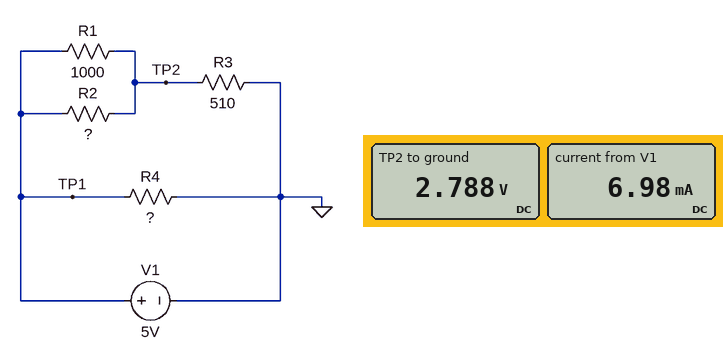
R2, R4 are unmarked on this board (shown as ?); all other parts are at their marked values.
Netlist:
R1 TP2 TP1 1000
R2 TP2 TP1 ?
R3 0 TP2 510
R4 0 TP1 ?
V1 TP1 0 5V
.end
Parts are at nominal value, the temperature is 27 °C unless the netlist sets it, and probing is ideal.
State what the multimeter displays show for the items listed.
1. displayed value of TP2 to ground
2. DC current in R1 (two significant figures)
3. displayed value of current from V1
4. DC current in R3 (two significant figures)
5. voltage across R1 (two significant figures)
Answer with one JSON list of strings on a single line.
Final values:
["2.788 V", "2.2 mA", "6.98 mA", "5.5 mA", "2.2 V"]
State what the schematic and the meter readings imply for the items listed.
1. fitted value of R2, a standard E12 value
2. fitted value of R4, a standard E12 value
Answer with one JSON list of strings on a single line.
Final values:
["680 Ω", "3.3 kΩ"]
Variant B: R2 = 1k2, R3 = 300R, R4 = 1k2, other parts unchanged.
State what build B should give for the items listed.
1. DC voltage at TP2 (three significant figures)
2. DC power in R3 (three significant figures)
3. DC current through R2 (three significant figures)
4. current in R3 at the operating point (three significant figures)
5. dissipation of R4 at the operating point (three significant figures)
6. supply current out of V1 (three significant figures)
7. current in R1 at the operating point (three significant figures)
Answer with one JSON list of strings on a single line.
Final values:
["1.77 V", "10.5 mW", "2.69 mA", "5.91 mA", "20.8 mW", "10.1 mA", "3.23 mA"]
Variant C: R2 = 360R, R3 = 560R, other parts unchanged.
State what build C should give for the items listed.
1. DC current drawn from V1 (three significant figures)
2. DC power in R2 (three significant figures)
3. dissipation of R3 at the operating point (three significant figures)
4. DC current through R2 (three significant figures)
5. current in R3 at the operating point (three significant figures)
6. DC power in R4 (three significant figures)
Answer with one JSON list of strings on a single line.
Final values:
["7.58 mA", "7.15 mW", "20.6 mW", "4.46 mA", "6.06 mA", "7.58 mW"]
